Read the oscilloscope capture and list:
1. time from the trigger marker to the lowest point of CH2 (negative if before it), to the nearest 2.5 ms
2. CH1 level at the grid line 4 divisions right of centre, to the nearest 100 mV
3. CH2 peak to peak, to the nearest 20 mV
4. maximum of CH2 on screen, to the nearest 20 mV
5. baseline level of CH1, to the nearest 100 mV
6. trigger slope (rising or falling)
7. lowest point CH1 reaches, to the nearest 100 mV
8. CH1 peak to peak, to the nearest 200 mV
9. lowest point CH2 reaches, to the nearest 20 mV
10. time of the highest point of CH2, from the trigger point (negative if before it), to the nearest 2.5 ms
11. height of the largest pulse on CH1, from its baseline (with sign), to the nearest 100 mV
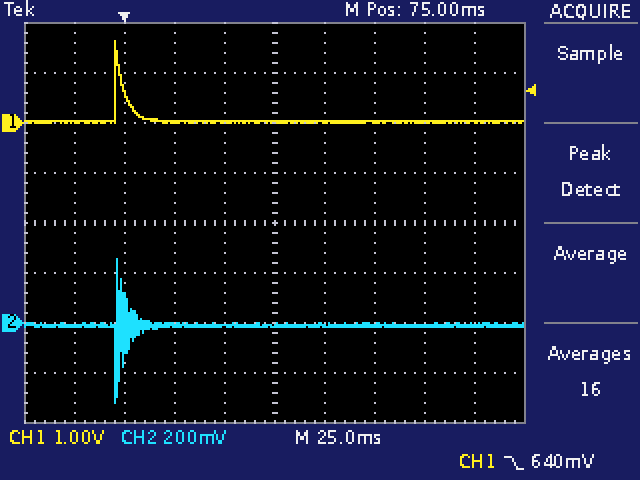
-5.0 ms
0.0 V
580 mV
260 mV
0.0 V
falling
0.0 V
1.6 V
-320 mV
-2.5 ms
+1.6 V
